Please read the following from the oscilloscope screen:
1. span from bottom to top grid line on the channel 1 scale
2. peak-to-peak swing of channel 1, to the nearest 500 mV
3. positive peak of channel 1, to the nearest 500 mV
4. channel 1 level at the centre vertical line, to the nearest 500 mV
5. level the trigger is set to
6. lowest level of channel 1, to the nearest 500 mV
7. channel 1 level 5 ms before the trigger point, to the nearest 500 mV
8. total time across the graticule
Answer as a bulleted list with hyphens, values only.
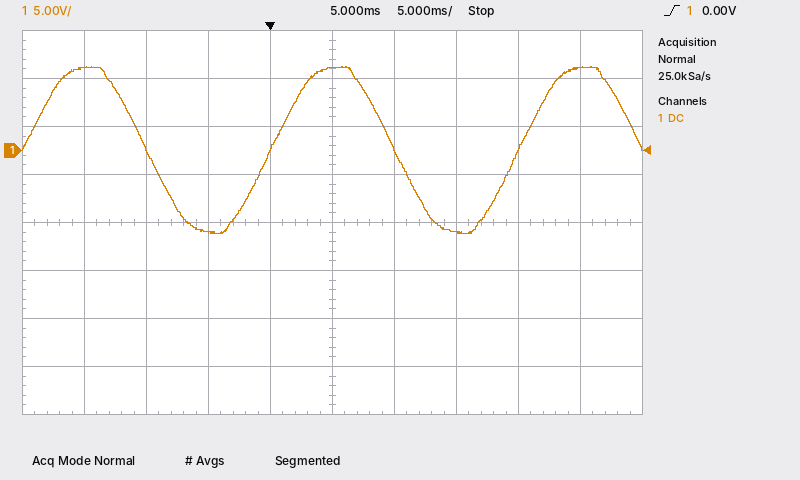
- 40 V
- 17.5 V
- 9.0 V
- 8.5 V
- 0.00 V
- -8.5 V
- -8.5 V
- 50 ms
